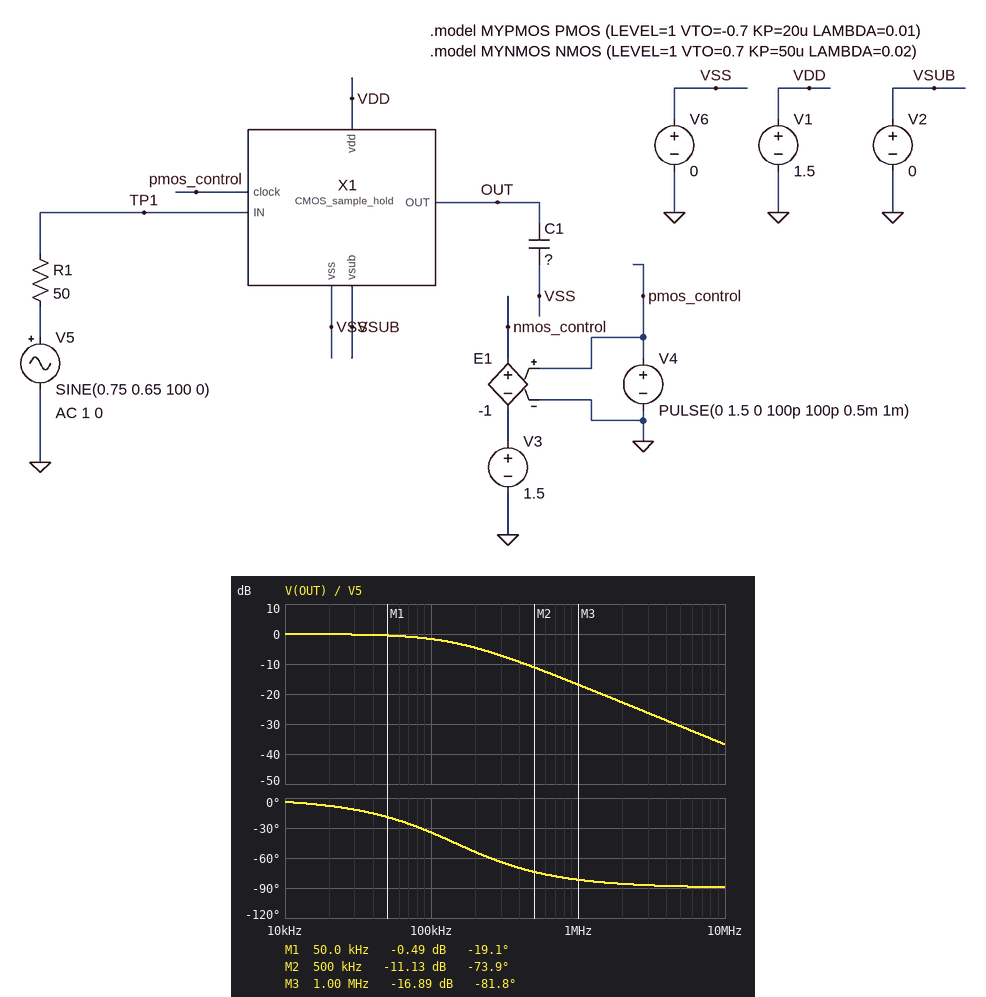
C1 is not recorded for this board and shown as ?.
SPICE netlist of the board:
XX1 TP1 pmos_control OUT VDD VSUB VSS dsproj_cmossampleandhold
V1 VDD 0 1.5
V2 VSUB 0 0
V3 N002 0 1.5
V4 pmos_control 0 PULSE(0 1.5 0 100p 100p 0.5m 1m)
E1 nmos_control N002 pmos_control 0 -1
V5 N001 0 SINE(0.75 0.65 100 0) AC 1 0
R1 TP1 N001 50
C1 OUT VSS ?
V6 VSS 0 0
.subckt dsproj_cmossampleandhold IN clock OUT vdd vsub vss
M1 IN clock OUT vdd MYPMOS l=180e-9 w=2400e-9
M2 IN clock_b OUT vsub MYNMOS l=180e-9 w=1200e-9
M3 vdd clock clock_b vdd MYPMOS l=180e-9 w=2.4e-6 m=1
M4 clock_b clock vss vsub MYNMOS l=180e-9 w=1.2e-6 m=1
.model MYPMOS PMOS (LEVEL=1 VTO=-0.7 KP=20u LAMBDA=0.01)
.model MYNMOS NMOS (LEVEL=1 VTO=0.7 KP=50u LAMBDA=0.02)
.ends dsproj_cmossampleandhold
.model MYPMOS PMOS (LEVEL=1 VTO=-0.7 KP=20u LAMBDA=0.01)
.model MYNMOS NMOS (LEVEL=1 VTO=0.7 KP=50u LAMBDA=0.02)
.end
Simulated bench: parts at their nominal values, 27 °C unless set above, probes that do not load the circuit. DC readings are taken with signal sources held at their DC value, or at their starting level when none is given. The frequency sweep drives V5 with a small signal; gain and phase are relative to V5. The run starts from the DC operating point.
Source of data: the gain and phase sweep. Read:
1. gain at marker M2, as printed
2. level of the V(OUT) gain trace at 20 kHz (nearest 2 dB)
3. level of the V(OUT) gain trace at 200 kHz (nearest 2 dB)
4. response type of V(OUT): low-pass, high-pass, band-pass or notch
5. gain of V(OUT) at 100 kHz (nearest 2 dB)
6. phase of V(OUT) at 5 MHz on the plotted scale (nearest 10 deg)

-11.13 dB
0 dB
-4 dB
low-pass
-2 dB
-90 deg
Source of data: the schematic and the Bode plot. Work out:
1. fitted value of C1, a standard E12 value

33 pF
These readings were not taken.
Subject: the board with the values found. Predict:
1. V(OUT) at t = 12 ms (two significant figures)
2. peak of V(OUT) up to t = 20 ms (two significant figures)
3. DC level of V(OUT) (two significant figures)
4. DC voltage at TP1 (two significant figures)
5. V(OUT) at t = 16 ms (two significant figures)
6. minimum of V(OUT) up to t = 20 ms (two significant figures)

1.4 V
1.4 V
750 mV
750 mV
370 mV
100 mV
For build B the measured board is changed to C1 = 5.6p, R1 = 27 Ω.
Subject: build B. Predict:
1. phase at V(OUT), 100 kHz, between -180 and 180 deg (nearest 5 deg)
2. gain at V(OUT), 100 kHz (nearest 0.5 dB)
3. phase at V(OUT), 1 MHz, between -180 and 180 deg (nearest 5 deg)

-5 deg
0 dB
-50 deg
